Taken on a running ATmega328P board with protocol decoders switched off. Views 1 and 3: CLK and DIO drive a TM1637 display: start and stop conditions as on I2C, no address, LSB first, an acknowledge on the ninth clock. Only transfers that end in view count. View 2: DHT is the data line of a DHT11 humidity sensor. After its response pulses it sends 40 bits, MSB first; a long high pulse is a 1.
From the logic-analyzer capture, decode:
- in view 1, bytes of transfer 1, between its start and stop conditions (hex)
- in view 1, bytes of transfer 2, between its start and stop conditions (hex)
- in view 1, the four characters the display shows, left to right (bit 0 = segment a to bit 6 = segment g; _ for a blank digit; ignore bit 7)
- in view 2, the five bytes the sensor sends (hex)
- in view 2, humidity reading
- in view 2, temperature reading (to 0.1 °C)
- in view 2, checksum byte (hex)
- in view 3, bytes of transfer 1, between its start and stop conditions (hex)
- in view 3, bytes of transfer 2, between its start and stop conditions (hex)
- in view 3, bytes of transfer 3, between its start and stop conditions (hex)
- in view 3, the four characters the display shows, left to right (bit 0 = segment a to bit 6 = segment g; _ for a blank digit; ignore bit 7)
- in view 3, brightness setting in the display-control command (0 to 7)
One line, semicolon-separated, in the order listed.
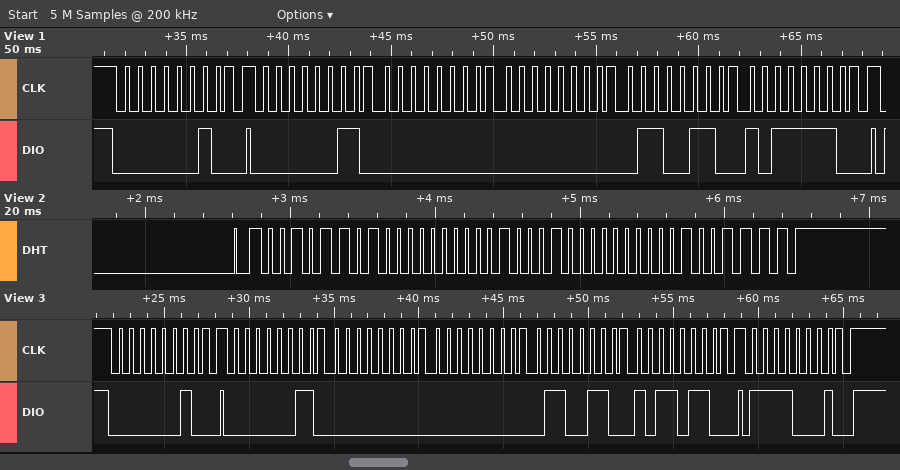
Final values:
40; C0 00 00 66 7D; __46; 2D 00 22 00 4F; 45 %; 34.0 °C; 0x4F; 40; C0 00 00 66 6D; 8F; __45; 7
